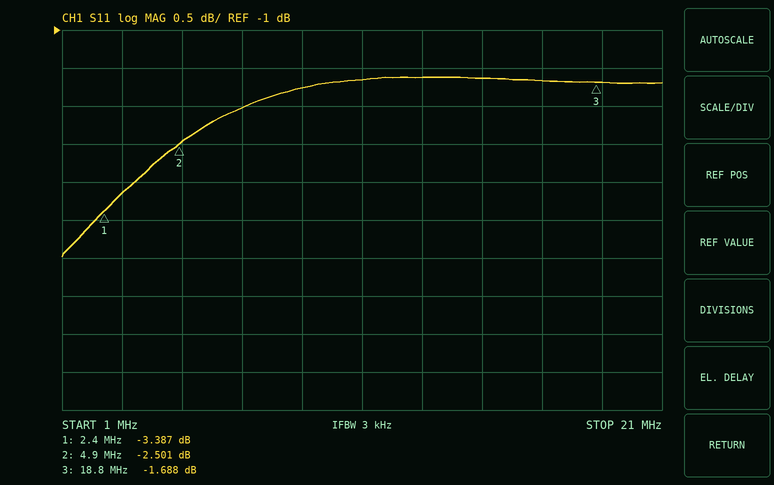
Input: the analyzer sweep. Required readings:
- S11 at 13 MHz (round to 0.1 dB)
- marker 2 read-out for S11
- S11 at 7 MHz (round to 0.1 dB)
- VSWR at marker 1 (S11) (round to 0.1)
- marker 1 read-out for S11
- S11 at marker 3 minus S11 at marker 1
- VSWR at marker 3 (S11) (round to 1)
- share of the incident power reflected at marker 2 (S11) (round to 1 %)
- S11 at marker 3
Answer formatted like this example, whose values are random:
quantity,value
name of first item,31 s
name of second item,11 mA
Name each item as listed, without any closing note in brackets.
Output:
quantity,value
S11 at 13 MHz,-1.6 dB
marker 2 read-out for S11,-2.501 dB
S11 at 7 MHz,-2.0 dB
VSWR at marker 1 (S11),5.2
marker 1 read-out for S11,-3.387 dB
S11 at marker 3 minus S11 at marker 1,1.699 dB
VSWR at marker 3 (S11),10
share of the incident power reflected at marker 2 (S11),56 %
S11 at marker 3,-1.688 dB
